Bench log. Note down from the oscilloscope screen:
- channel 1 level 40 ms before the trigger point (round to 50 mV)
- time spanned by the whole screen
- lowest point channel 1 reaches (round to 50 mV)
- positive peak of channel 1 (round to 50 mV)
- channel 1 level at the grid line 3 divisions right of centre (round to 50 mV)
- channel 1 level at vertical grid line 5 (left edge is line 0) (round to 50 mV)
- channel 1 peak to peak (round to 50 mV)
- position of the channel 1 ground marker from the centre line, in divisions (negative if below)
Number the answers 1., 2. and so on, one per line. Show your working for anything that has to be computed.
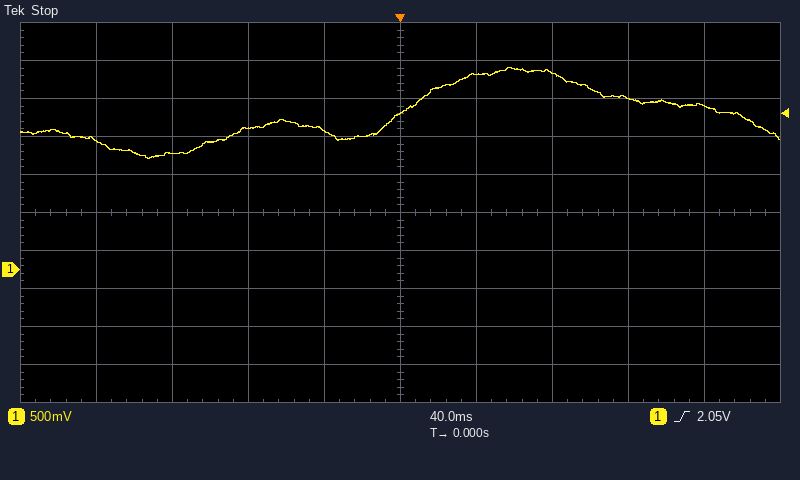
1. 1.85 V
2. 400 ms
3. 1.45 V
4. 2.65 V
5. 2.25 V
6. 2.05 V
7. 2.65 V − (1.45 V) = 1.20 V
8. -1.5 div
